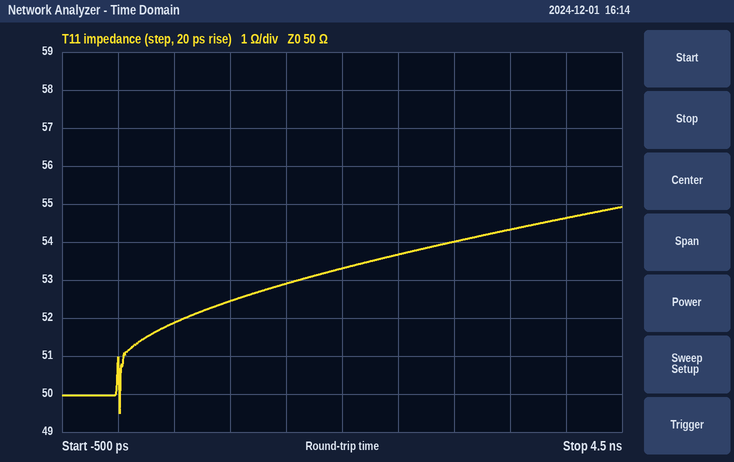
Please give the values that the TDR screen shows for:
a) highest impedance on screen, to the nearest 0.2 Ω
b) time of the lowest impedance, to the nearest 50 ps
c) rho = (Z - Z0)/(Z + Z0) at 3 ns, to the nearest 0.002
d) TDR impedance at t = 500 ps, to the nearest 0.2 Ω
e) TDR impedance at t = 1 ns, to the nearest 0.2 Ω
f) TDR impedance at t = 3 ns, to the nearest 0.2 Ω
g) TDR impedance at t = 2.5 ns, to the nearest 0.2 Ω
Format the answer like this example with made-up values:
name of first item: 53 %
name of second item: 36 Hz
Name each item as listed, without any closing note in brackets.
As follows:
highest impedance on screen, to the nearest 0.2 Ω: 55.0 Ω
time of the lowest impedance, to the nearest 50 ps: 0 ps
rho = (Z - Z0)/(Z + Z0) at 3 ns, to the nearest 0.002: +0.038
TDR impedance at t = 500 ps, to the nearest 0.2 Ω: 51.8 Ω
TDR impedance at t = 1 ns, to the nearest 0.2 Ω: 52.4 Ω
TDR impedance at t = 3 ns, to the nearest 0.2 Ω: 54.0 Ω
TDR impedance at t = 2.5 ns, to the nearest 0.2 Ω: 53.6 Ω
